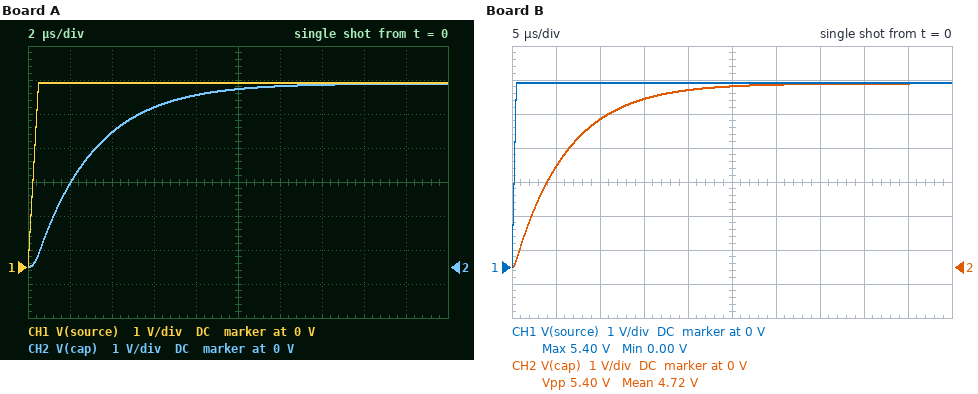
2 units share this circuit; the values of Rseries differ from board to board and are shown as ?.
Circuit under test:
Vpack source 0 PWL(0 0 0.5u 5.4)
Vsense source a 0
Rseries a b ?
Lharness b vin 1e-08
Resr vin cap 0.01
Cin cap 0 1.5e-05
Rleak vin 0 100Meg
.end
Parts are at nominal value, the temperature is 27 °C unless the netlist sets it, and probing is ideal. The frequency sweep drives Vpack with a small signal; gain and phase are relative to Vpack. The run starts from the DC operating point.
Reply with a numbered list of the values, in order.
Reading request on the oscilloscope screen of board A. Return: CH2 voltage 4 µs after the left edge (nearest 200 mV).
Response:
1. 4.0 V
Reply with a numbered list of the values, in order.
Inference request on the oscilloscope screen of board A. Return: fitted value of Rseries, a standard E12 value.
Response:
1. 0.18 Ω
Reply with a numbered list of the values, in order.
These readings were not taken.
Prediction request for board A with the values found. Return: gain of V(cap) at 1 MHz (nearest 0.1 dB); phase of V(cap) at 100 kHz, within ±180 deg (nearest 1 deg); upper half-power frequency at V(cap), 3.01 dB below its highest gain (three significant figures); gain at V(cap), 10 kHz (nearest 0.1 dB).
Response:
1. -25.4 dB
2. -62 deg
3. 56.9 kHz
4. -0.1 dB
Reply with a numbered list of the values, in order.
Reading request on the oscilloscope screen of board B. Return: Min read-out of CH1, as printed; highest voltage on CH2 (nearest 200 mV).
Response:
1. 0.00 V
2. 5.4 V
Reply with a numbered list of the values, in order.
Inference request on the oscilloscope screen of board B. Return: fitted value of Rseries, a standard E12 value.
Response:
1. 0.39 Ω
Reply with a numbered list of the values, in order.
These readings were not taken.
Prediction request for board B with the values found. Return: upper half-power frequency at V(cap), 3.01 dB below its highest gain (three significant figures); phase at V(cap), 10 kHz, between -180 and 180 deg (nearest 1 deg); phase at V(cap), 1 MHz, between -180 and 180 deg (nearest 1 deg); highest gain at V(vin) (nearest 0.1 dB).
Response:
1. 26.6 kHz
2. -21 deg
3. -97 deg
4. 0 dB
